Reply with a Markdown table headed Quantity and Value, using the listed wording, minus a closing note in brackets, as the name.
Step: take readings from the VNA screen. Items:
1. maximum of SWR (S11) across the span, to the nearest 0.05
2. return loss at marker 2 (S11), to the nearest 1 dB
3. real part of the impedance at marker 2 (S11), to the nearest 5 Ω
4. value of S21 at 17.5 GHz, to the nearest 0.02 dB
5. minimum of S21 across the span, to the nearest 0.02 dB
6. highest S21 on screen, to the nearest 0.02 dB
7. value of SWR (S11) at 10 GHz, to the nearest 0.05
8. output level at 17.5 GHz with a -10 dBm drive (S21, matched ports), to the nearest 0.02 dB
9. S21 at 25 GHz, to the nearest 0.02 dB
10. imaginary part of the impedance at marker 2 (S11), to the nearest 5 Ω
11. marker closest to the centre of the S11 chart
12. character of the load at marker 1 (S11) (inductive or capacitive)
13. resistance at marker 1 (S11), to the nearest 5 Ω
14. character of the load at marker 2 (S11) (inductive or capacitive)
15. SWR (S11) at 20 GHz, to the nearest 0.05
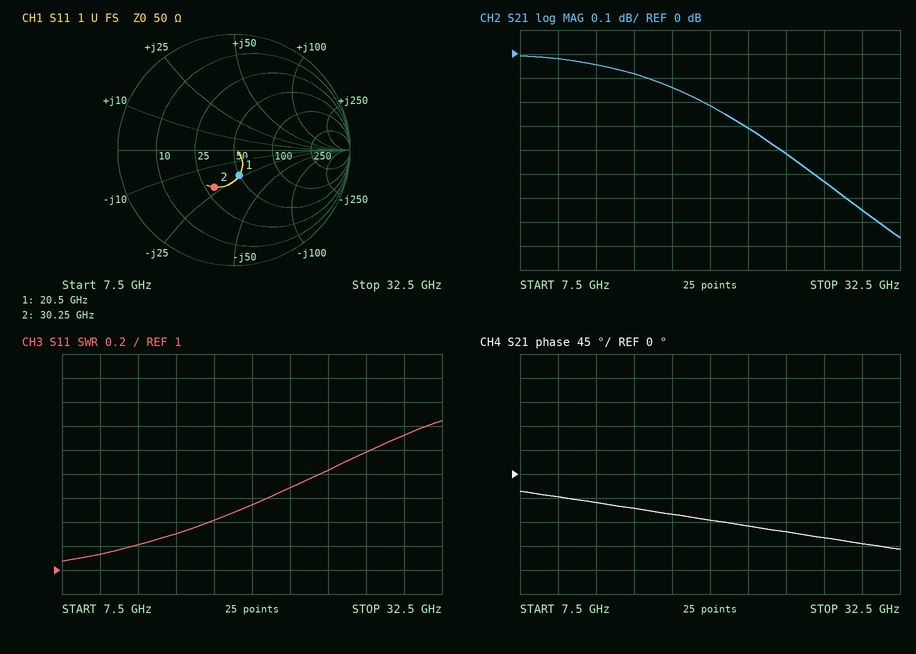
| Quantity | Value |
|---|---|
| maximum of SWR (S11) across the span, to the nearest 0.05 | 2.25 |
| return loss at marker 2 (S11), to the nearest 1 dB | 9 dB |
| real part of the impedance at marker 2 (S11), to the nearest 5 Ω | 30 Ω |
| value of S21 at 17.5 GHz, to the nearest 0.02 dB | -0.14 dB |
| minimum of S21 across the span, to the nearest 0.02 dB | -0.76 dB |
| highest S21 on screen, to the nearest 0.02 dB | 0.00 dB |
| value of SWR (S11) at 10 GHz, to the nearest 0.05 | 1.15 |
| output level at 17.5 GHz with a -10 dBm drive (S21, matched ports), to the nearest 0.02 dB | -10.14 dBm |
| S21 at 25 GHz, to the nearest 0.02 dB | -0.42 dB |
| imaginary part of the impedance at marker 2 (S11), to the nearest 5 Ω | -20 Ω |
| marker closest to the centre of the S11 chart | marker 1 |
| character of the load at marker 1 (S11) | capacitive |
| resistance at marker 1 (S11), to the nearest 5 Ω | 50 Ω |
| character of the load at marker 2 (S11) | capacitive |
| SWR (S11) at 20 GHz, to the nearest 0.05 | 1.55 |
